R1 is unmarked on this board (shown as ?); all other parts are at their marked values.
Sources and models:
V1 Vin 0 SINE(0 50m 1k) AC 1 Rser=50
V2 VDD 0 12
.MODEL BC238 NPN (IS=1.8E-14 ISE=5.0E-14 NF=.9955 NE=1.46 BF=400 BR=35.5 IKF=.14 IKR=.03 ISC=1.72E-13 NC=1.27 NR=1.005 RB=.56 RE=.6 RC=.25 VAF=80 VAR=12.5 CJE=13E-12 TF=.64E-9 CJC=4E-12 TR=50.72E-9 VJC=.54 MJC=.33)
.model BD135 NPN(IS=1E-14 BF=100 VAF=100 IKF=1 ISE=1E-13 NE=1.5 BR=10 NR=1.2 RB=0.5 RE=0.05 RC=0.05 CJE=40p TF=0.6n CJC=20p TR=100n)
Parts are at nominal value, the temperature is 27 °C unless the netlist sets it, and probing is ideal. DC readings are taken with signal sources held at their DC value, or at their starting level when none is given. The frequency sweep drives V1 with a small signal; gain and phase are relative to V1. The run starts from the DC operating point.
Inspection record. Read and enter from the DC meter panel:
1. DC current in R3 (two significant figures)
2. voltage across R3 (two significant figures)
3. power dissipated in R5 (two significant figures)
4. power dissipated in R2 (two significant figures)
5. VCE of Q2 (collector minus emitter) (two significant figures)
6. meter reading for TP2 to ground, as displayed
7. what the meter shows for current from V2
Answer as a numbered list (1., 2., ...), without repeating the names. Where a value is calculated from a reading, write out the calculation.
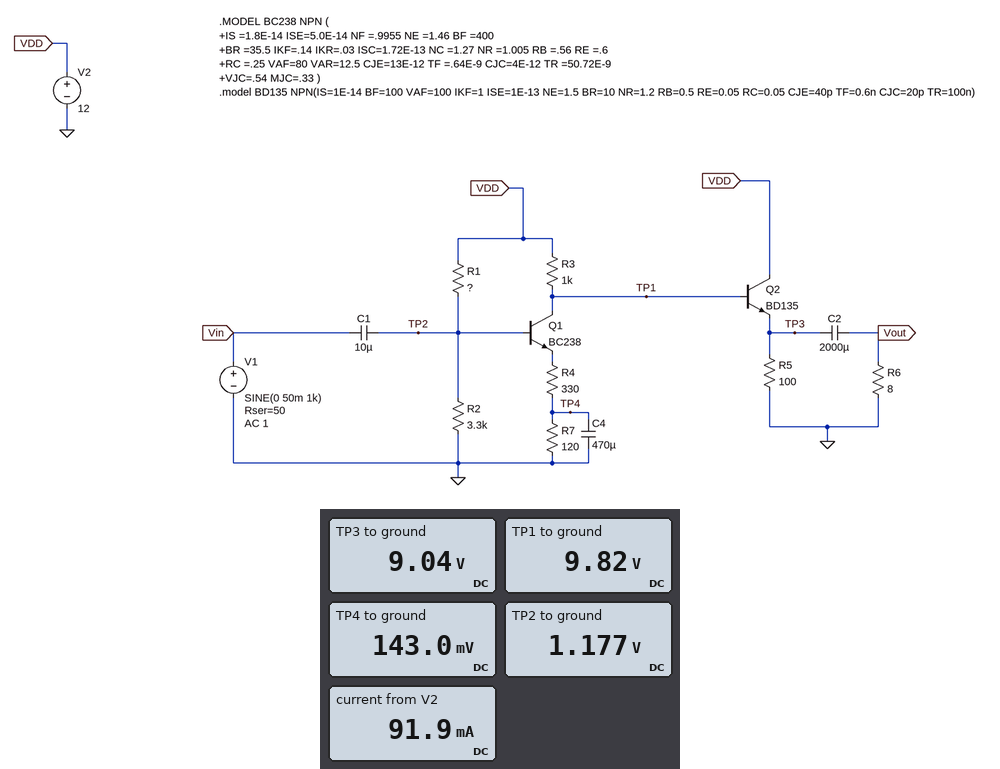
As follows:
1. (12 V - 9.82 V) / 1 kΩ = 2.2 mA
2. 12 V - 9.82 V = 2.2 V
3. (9.04 V)^2 / 100 Ω = 820 mW
4. (1.177 V)^2 / 3.3 kΩ = 420 µW
5. 12 V - 9.04 V = 3.0 V
6. 1.177 V
7. 91.9 mA
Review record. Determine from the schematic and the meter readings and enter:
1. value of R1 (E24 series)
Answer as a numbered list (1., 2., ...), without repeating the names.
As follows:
1. 30 kΩ
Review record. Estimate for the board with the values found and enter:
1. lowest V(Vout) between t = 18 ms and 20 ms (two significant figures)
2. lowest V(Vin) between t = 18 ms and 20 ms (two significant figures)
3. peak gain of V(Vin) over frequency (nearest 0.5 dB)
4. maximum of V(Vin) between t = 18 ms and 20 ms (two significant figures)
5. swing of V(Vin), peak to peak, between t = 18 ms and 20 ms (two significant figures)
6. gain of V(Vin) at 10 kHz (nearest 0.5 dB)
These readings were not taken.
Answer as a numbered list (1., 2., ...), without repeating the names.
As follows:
1. -53 mV
2. -49 mV
3. 0 dB
4. 49 mV
5. 98 mV
6. 0 dB
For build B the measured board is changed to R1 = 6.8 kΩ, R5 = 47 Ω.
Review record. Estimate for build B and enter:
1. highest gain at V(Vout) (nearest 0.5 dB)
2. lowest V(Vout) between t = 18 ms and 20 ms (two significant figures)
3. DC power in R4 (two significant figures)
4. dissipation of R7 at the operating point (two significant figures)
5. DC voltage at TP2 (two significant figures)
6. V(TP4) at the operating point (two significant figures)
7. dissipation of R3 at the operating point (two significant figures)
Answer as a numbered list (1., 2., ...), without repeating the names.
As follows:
1. 1.0 dB
2. -55 mV
3. 16 mW
4. 6.0 mW
5. 3.9 V
6. 850 mV
7. 61 mW
